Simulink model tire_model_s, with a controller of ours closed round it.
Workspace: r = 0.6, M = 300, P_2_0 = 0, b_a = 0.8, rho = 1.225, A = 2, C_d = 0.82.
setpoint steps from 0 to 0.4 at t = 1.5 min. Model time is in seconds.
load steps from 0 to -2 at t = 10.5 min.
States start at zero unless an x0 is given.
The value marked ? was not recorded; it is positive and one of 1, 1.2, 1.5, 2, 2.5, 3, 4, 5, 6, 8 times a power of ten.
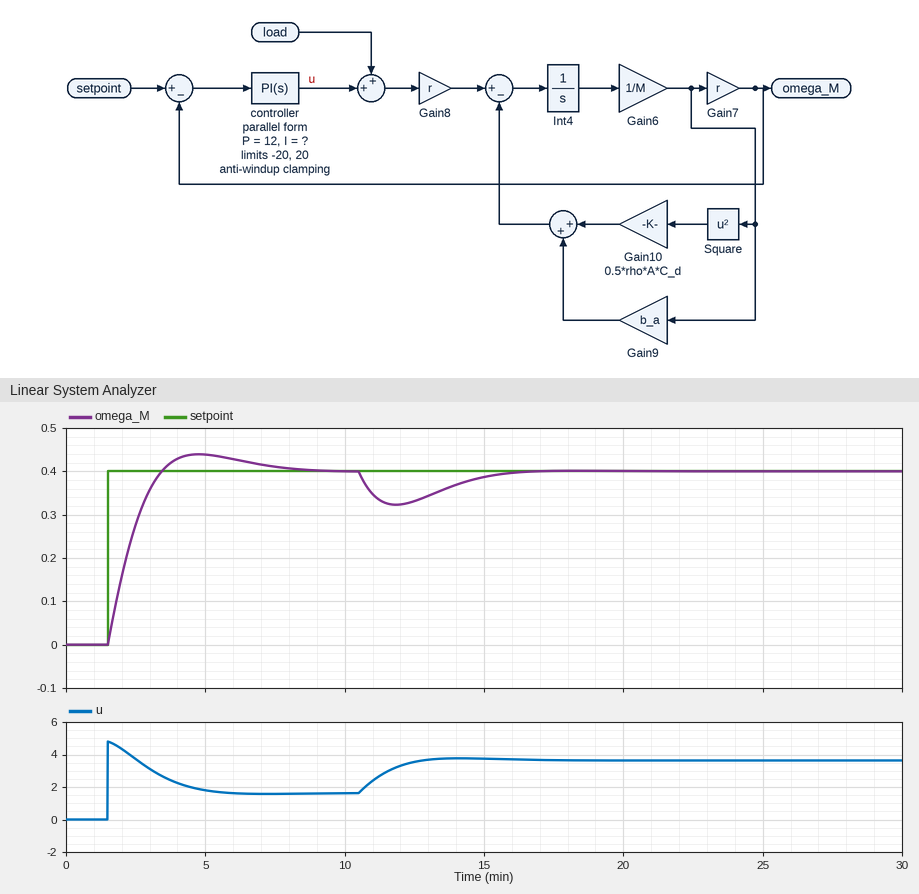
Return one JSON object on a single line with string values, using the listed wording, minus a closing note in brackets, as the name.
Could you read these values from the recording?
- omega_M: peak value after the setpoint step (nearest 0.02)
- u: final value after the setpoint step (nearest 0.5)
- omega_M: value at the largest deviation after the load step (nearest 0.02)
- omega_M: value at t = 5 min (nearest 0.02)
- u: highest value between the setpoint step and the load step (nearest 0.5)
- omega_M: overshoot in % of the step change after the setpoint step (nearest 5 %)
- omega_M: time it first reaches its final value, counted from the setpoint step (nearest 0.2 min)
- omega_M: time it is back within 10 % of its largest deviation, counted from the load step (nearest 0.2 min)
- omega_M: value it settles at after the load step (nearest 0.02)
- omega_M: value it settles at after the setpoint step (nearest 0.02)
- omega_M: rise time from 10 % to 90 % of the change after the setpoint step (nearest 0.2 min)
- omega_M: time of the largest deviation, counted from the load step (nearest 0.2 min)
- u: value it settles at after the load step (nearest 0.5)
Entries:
{"omega_M: peak value after the setpoint step": "0.44", "u: final value after the setpoint step": "1.5", "omega_M: value at the largest deviation after the load step": "0.32", "omega_M: value at t = 5 min": "0.44", "u: highest value between the setpoint step and the load step": "5.0", "omega_M: overshoot in % of the step change after the setpoint step": "10 %", "omega_M: time it first reaches its final value, counted from the setpoint step": "2.0 min", "omega_M: time it is back within 10 % of its largest deviation, counted from the load step": "5.0 min", "omega_M: value it settles at after the load step": "0.40", "omega_M: value it settles at after the setpoint step": "0.40", "omega_M: rise time from 10 % to 90 % of the change after the setpoint step": "1.4 min", "omega_M: time of the largest deviation, counted from the load step": "1.4 min", "u: value it settles at after the load step": "3.5"}
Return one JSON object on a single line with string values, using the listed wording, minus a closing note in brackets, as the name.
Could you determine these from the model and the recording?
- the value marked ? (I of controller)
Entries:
{"the value marked ?": "0.15"}
